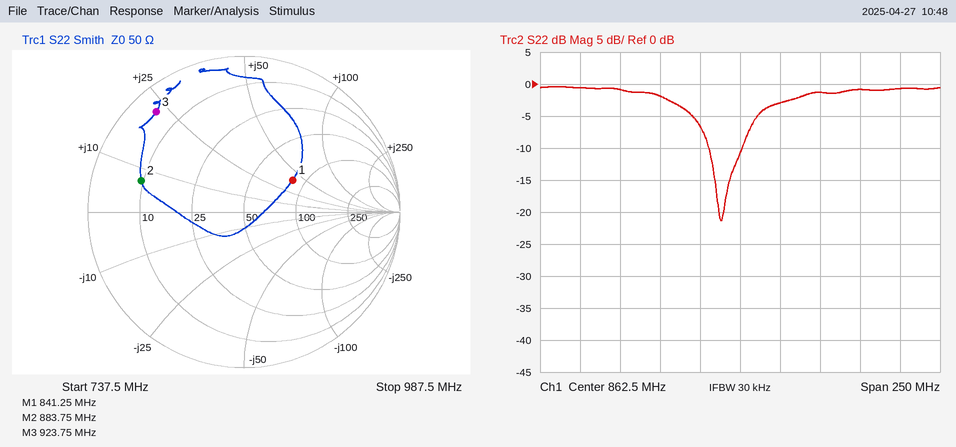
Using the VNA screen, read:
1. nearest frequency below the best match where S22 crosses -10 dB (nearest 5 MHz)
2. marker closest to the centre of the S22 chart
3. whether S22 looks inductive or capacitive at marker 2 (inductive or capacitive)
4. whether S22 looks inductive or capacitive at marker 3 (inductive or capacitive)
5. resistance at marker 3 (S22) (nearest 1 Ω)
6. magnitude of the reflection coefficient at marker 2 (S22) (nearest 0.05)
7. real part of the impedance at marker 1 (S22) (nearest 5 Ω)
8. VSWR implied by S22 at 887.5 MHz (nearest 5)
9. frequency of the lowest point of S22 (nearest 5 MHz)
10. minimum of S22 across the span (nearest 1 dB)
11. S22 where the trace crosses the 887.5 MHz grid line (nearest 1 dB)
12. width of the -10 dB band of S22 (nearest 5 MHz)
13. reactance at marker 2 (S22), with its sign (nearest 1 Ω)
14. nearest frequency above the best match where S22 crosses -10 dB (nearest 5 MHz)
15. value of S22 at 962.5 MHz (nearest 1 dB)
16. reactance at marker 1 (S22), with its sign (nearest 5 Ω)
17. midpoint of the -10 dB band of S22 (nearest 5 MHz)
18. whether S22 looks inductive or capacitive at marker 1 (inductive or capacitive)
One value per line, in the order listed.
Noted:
845 MHz
marker 1
inductive
inductive
5 Ω
0.70
85 Ω
5
850 MHz
-21 dB
-3 dB
20 MHz
+7 Ω
865 MHz
-1 dB
+40 Ω
855 MHz
inductive
